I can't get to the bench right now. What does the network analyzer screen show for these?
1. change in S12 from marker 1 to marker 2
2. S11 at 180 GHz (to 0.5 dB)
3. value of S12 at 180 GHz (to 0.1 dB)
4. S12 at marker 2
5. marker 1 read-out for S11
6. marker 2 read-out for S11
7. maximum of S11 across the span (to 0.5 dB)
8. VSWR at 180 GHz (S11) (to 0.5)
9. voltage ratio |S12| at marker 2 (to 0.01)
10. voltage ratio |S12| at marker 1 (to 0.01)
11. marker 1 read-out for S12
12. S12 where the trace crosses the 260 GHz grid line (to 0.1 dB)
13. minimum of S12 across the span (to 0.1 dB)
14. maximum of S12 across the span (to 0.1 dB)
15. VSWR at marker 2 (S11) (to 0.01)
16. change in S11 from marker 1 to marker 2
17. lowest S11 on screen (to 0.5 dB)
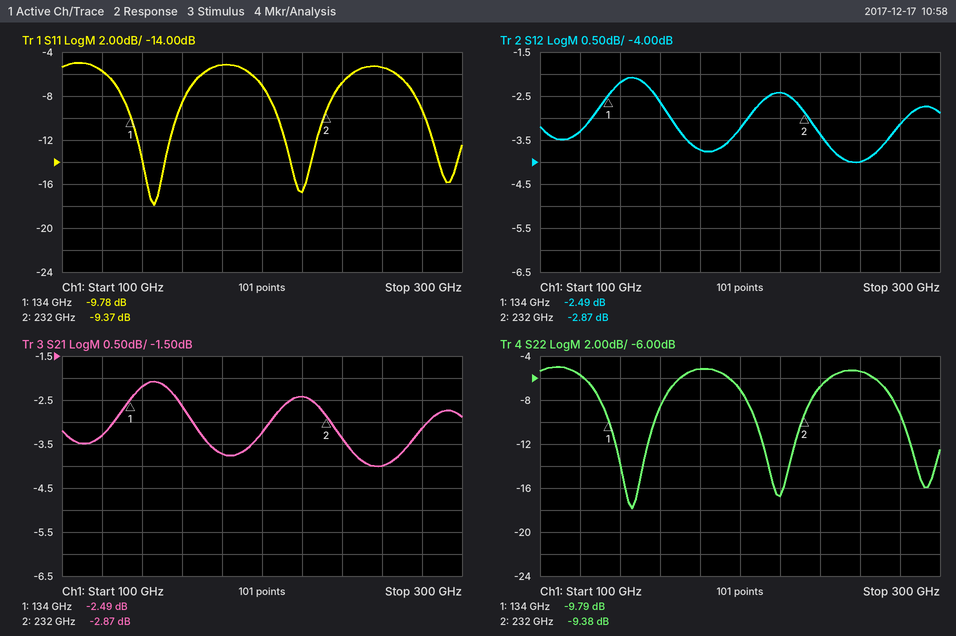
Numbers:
-0.38 dB
-5.0 dB
-3.7 dB
-2.87 dB
-9.78 dB
-9.37 dB
-5.0 dB
3.5
0.72
0.75
-2.49 dB
-4.0 dB
-4.0 dB
-2.1 dB
2.03
0.41 dB
-18.0 dB
